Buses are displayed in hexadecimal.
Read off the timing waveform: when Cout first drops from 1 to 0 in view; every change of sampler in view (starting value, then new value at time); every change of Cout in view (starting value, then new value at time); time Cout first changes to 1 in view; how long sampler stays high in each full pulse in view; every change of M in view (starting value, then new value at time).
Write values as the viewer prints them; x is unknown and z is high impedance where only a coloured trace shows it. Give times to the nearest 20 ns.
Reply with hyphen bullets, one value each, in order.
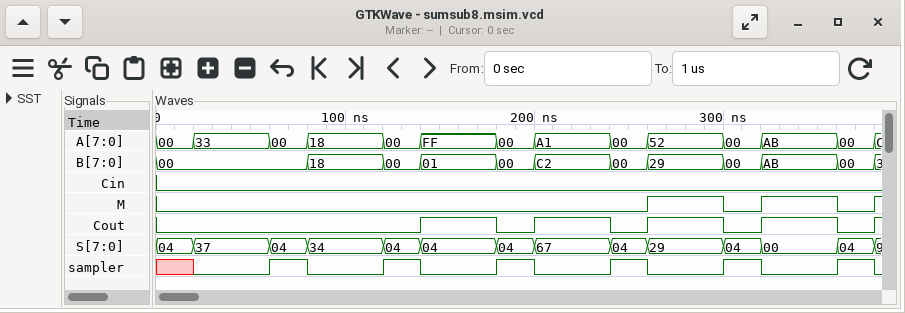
- 180 ns
- x, 0 at 20 ns, 1 at 60 ns, 0 at 80 ns, 1 at 120 ns, 0 at 140 ns, 1 at 180 ns, 0 at 200 ns, 1 at 240 ns, 0 at 260 ns, 1 at 300 ns, 0 at 320 ns, 1 at 360 ns, 0 at 380 ns
- 0, 1 at 140 ns, 0 at 180 ns, 1 at 200 ns, 0 at 240 ns, 1 at 260 ns, 0 at 300 ns, 1 at 320 ns, 0 at 360 ns, 1 at 380 ns
- 140 ns
- 20 ns, 20 ns, 20 ns, 20 ns, 20 ns, 20 ns
- 0, 1 at 260 ns, 0 at 300 ns, 1 at 320 ns, 0 at 360 ns, 1 at 380 ns
